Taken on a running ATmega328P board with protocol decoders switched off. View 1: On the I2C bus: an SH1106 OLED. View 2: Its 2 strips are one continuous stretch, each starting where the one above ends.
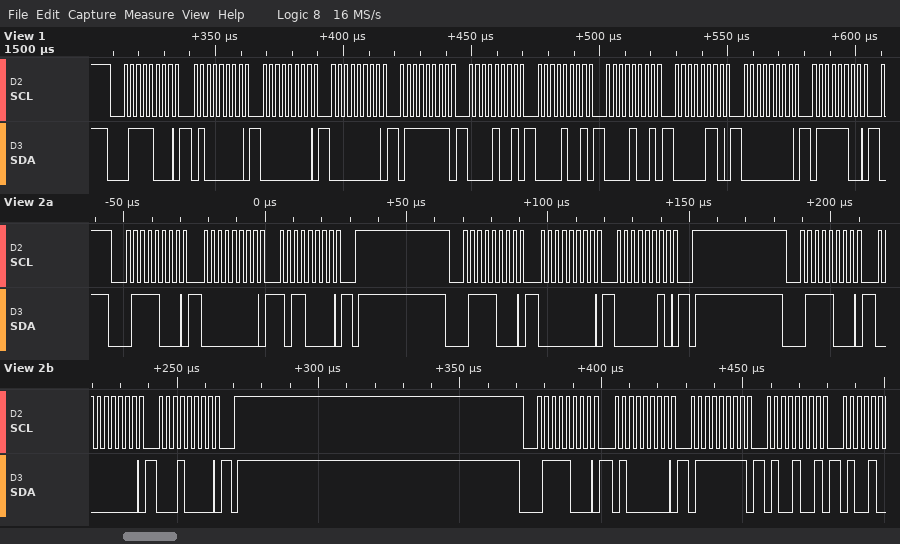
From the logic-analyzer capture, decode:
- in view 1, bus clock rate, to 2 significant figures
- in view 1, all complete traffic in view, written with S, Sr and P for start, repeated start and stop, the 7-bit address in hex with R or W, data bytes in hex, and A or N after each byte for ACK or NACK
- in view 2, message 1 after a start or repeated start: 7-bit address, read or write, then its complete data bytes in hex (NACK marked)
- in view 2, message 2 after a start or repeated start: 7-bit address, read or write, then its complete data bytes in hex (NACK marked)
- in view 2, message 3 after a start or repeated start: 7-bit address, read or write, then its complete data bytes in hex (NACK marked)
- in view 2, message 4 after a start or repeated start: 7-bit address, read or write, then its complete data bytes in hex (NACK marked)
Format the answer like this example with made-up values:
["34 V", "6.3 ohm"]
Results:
["400 kHz", "S 3CW A 40 A 00 A 00 A 7F A 09 A 09 A 09 A 06 A 00 A 7C A", "0x3C write: 00 B0", "0x3C write: 00 02", "0x3C write: 00 10", "0x3C write: 40 7F 49"]
